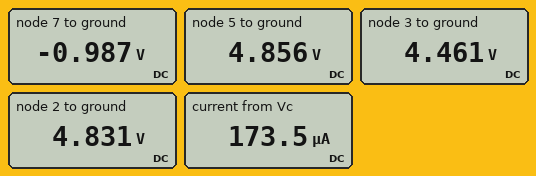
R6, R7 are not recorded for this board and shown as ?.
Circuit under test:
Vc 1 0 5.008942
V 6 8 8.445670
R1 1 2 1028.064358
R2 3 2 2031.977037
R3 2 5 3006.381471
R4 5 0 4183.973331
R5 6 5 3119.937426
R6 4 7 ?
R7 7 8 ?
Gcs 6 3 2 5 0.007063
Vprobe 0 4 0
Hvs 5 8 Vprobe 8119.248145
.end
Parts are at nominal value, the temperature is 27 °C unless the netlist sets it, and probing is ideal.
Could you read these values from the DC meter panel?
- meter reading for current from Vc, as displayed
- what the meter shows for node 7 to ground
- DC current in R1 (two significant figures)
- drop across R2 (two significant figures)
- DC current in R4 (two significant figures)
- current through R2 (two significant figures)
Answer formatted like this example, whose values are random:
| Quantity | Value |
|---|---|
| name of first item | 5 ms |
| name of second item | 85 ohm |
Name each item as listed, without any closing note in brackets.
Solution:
| Quantity | Value |
|---|---|
| meter reading for current from Vc, as displayed | 173.5 µA |
| what the meter shows for node 7 to ground | -0.987 V |
| DC current in R1 | 170 µA |
| drop across R2 | 370 mV |
| DC current in R4 | 1.2 mA |
| current through R2 | 180 µA |
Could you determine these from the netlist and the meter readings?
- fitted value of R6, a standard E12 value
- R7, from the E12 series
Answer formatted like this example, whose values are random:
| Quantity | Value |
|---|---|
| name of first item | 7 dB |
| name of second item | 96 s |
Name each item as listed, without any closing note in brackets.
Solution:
| Quantity | Value |
|---|---|
| fitted value of R6, a standard E12 value | 1 kΩ |
| R7, from the E12 series | 2.2 kΩ |
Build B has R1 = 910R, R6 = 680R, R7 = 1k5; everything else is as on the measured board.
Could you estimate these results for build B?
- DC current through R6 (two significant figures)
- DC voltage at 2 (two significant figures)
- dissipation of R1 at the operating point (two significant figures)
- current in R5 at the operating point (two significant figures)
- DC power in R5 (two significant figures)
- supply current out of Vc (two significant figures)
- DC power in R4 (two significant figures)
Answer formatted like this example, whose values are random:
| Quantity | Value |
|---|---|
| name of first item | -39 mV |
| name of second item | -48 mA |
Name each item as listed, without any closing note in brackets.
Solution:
| Quantity | Value |
|---|---|
| DC current through R6 | 800 µA |
| DC voltage at 2 | 4.7 V |
| dissipation of R1 at the operating point | 100 µW |
| current in R5 at the operating point | 620 µA |
| DC power in R5 | 1.2 mW |
| supply current out of Vc | 340 µA |
| DC power in R4 | 5.4 mW |
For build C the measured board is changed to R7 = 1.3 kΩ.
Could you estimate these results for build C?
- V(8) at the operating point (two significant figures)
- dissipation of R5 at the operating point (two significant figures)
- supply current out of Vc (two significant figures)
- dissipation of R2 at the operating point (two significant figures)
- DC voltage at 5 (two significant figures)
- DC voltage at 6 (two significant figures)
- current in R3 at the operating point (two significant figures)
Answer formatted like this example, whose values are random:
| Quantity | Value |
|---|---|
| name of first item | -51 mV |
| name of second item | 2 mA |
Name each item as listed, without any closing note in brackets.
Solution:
| Quantity | Value |
|---|---|
| V(8) at the operating point | -1.9 V |
| dissipation of R5 at the operating point | 1.1 mW |
| supply current out of Vc | 320 µA |
| dissipation of R2 at the operating point | 230 µW |
| DC voltage at 5 | 4.7 V |
| DC voltage at 6 | 6.6 V |
| current in R3 at the operating point | 16 µA |
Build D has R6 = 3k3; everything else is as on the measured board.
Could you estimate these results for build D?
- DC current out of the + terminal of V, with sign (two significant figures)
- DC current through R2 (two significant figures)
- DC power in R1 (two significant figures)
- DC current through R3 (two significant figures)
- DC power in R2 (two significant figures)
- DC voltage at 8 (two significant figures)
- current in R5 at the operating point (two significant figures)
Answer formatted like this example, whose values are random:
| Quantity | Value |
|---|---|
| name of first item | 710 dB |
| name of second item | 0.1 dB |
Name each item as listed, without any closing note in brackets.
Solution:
| Quantity | Value |
|---|---|
| DC current out of the + terminal of V, with sign | -2.1 mA |
| DC current through R2 | 860 µA |
| DC power in R1 | 690 µW |
| DC current through R3 | 40 µA |
| DC power in R2 | 1.5 mW |
| DC voltage at 8 | -12 V |
| current in R5 at the operating point | 3.0 mA |
